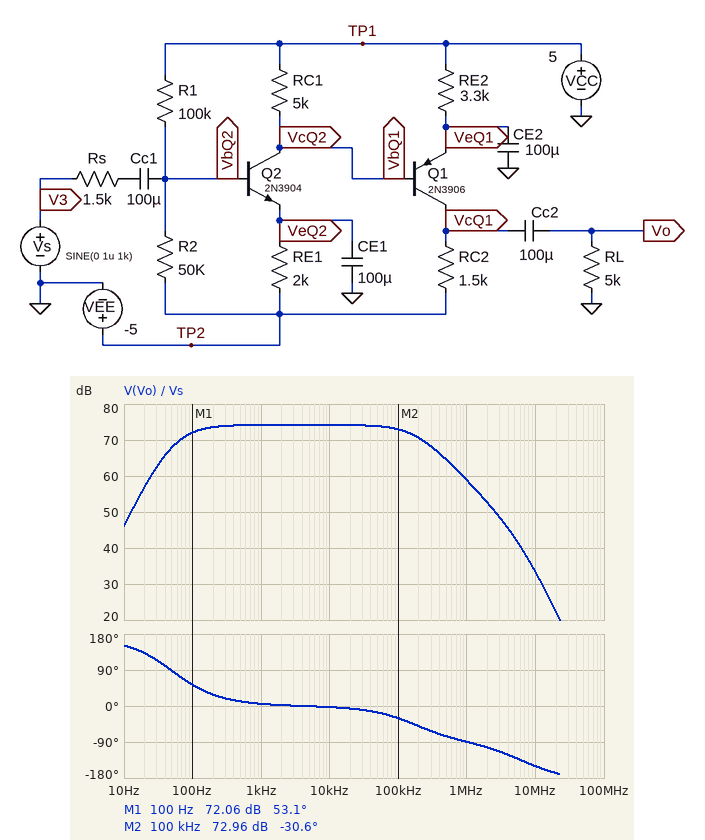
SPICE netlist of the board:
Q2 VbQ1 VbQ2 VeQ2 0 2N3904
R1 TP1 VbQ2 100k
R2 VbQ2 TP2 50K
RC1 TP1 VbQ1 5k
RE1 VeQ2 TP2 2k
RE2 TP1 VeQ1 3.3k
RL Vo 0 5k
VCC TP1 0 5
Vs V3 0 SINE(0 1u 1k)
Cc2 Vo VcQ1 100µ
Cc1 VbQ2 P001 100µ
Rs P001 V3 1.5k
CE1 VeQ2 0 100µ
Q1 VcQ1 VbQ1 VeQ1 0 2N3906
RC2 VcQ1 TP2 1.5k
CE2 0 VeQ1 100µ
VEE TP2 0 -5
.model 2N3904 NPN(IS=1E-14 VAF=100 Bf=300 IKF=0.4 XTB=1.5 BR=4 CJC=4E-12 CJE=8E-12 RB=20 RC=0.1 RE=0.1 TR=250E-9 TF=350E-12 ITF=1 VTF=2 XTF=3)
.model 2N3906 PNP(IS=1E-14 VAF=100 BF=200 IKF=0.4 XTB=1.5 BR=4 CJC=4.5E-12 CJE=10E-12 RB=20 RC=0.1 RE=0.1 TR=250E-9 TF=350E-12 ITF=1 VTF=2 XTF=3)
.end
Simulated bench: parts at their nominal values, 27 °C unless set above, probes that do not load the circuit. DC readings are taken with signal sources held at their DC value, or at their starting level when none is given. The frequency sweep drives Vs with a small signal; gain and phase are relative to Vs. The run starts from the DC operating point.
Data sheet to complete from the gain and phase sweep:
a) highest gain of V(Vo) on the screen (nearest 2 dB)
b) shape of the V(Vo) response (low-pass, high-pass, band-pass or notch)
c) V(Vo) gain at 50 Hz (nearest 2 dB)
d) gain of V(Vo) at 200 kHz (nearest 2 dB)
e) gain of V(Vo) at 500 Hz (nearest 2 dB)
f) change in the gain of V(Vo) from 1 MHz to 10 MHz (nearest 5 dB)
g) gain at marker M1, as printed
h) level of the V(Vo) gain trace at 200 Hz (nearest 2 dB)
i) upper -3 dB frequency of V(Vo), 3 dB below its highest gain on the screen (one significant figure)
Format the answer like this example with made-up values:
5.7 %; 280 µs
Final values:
74 dB; band-pass; 68 dB; 70 dB; 74 dB; -25 dB; 72.06 dB; 74 dB; 200 kHz
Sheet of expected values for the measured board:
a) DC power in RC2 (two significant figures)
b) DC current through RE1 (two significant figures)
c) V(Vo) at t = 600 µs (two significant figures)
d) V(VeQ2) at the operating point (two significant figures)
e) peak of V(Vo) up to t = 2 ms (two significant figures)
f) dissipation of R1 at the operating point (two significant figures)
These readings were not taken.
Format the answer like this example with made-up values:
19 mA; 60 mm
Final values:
4.3 mW; 1.3 mA; -3.7 mV; -2.5 V; 4.8 mV; 460 µW
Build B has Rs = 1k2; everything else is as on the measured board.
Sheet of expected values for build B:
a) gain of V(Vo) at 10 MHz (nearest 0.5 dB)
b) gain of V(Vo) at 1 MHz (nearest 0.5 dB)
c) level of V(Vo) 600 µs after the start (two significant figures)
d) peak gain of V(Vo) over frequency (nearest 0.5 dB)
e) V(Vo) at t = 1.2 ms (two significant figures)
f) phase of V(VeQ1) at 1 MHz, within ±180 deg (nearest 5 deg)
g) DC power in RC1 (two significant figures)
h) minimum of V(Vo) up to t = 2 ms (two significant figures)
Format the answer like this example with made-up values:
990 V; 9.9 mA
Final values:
35.0 dB; 60.0 dB; -3.9 mV; 74.5 dB; 4.9 mV; 5 deg; 7.9 mW; -5.7 mV
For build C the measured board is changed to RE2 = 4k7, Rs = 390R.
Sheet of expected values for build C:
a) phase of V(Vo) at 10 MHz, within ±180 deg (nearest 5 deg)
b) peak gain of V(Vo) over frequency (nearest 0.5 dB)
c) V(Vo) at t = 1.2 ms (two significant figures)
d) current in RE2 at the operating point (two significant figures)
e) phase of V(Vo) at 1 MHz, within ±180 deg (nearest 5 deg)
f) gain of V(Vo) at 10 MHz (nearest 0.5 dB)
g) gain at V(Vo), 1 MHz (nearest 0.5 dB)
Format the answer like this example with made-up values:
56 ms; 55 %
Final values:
-125 deg; 74.5 dB; 4.9 mV; 1.2 mA; -80 deg; 41.5 dB; 63.0 dB
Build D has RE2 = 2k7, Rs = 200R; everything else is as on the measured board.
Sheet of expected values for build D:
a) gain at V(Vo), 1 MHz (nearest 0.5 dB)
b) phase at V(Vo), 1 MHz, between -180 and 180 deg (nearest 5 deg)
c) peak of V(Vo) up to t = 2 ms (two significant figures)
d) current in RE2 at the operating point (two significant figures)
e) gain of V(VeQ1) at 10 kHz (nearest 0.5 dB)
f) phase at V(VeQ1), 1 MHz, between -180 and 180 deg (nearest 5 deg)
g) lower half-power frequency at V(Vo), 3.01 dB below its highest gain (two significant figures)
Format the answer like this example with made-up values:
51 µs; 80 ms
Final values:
64.0 dB; -80 deg; 6.4 mV; 2.1 mA; -0.5 dB; 10 deg; 93 Hz
